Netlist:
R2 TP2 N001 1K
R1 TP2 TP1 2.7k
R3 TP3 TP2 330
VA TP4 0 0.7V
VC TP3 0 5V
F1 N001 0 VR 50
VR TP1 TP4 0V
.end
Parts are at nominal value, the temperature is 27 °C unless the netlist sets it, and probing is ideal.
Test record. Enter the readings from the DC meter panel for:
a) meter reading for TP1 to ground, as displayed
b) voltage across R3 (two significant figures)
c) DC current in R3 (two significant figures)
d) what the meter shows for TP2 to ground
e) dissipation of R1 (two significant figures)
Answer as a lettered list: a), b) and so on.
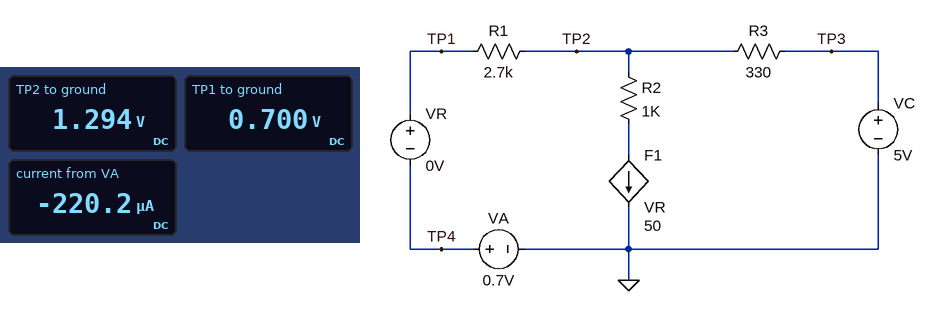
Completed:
a) 0.700 V
b) 3.7 V
c) 11 mA
d) 1.294 V
e) 130 µW
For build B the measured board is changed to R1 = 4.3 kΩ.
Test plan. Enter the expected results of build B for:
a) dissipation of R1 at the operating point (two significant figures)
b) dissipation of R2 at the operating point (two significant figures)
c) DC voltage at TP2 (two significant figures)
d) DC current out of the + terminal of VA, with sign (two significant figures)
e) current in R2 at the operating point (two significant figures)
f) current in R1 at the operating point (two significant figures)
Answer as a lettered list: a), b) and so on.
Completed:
a) 180 µW
b) 100 mW
c) 1.6 V
d) -200 µA
e) 10 mA
f) 200 µA
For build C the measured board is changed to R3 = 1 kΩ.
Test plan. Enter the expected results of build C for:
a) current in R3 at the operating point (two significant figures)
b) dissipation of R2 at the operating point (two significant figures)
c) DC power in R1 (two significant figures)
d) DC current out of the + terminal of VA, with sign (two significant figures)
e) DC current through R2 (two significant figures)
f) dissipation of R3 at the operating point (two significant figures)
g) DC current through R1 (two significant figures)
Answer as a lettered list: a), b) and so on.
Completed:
a) 4.1 mA
b) 16 mW
c) 17 µW
d) -80 µA
e) 4.0 mA
f) 17 mW
g) 80 µA
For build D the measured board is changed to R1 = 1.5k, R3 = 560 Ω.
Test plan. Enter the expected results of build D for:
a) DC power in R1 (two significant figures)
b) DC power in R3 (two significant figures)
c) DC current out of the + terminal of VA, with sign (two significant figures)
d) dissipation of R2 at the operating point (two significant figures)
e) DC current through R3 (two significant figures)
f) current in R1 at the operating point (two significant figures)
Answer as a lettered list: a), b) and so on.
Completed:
a) 31 µW
b) 30 mW
c) -140 µA
d) 51 mW
e) 7.3 mA
f) 140 µA
